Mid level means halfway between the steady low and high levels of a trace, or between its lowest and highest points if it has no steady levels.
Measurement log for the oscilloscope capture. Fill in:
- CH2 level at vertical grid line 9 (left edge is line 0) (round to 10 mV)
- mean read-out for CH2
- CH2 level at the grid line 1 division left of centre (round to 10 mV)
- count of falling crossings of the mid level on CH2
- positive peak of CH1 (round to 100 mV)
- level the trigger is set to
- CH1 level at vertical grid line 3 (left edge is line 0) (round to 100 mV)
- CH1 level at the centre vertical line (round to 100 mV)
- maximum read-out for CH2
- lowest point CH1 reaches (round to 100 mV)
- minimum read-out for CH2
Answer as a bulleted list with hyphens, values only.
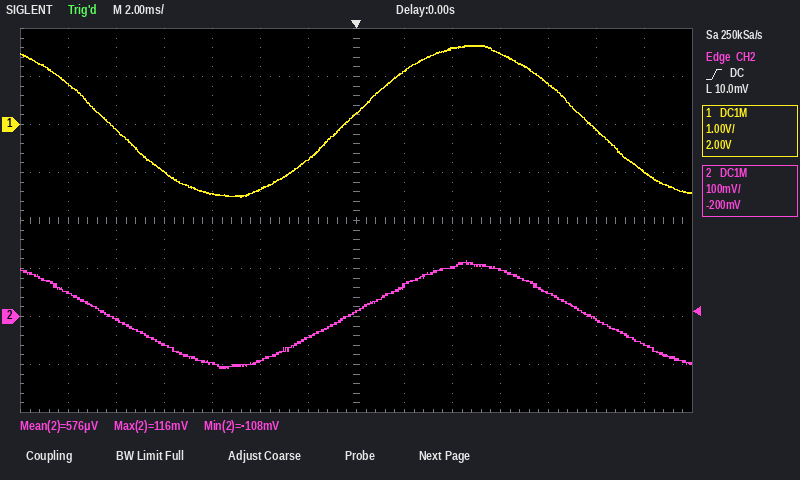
- 100 mV
- 576 µV
- -40 mV
- 2
- 1.6 V
- 10.0 mV
- -1.0 V
- 200 mV
- 116 mV
- -1.5 V
- -108 mV
